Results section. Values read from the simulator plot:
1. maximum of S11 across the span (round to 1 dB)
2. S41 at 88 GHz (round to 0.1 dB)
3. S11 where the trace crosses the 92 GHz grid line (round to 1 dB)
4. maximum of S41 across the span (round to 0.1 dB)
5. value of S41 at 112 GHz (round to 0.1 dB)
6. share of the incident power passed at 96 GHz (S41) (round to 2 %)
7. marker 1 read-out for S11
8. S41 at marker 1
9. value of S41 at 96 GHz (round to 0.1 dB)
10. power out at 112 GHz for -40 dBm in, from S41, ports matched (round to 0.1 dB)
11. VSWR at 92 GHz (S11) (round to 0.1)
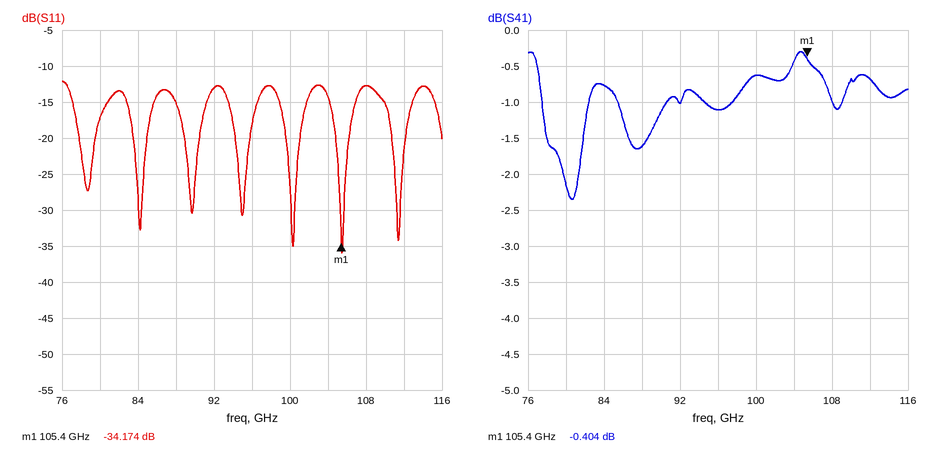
-12 dB
-1.6 dB
-13 dB
-0.3 dB
-0.7 dB
78 %
-34.174 dB
-0.404 dB
-1.1 dB
-40.7 dBm
1.6
